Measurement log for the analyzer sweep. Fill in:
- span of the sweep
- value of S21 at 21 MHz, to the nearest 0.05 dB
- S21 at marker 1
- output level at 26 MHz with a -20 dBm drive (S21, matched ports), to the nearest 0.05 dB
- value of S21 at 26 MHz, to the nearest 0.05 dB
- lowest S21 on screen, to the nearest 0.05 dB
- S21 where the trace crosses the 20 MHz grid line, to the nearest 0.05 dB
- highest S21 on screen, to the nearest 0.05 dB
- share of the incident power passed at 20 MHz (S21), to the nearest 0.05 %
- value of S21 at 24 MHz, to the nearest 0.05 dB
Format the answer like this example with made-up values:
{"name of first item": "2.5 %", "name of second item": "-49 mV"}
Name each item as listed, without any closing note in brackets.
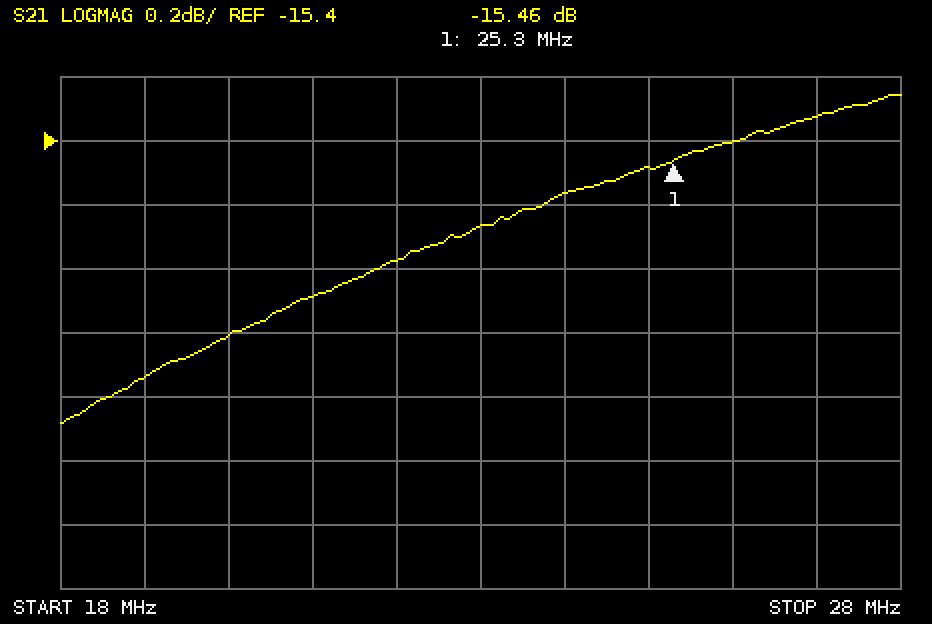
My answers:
{"span of the sweep": "10 MHz", "value of S21 at 21 MHz, to the nearest 0.05 dB": "-15.90 dB", "S21 at marker 1": "-15.46 dB", "output level at 26 MHz with a -20 dBm drive (S21, matched ports), to the nearest 0.05 dB": "-35.40 dBm", "value of S21 at 26 MHz, to the nearest 0.05 dB": "-15.40 dB", "lowest S21 on screen, to the nearest 0.05 dB": "-16.30 dB", "S21 where the trace crosses the 20 MHz grid line, to the nearest 0.05 dB": "-16.00 dB", "highest S21 on screen, to the nearest 0.05 dB": "-15.25 dB", "share of the incident power passed at 20 MHz (S21), to the nearest 0.05 %": "2.50 %", "value of S21 at 24 MHz, to the nearest 0.05 dB": "-15.55 dB"}
